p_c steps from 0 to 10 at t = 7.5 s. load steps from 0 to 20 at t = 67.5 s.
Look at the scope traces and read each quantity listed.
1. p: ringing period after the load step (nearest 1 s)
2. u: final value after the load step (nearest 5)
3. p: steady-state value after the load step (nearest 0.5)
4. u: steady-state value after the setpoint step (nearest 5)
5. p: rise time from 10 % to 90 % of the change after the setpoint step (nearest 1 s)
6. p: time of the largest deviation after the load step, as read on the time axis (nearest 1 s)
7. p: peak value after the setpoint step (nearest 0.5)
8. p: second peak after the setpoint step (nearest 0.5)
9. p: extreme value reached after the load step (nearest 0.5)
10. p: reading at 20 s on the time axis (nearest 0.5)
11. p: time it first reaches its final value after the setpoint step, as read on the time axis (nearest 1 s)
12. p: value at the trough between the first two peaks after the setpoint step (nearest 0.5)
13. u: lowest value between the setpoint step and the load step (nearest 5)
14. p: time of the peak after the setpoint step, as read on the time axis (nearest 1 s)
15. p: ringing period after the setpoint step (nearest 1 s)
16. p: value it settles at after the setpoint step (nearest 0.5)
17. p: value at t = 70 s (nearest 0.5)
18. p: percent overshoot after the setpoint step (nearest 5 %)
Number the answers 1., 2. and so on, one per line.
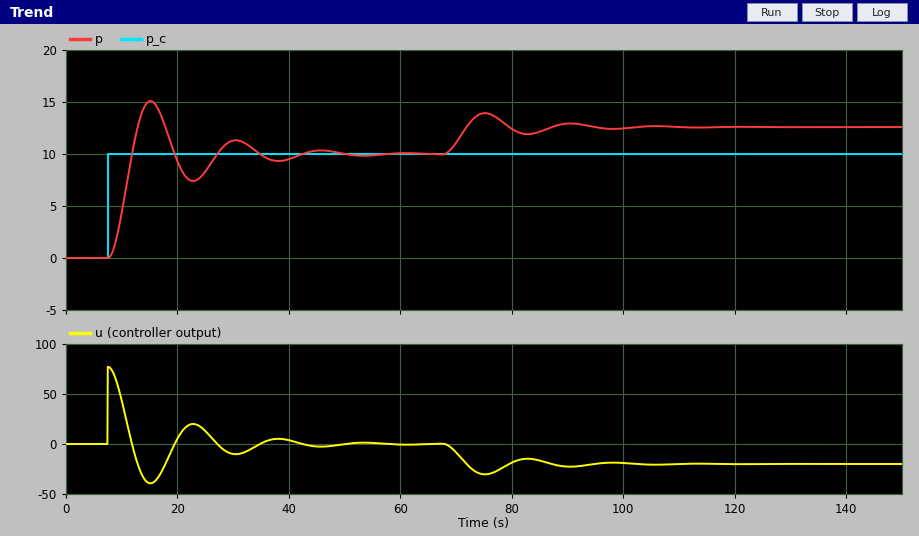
1. 15 s
2. -20
3. 12.5
4. 0
5. 3 s
6. 75 s
7. 15.0
8. 11.5
9. 14.0
10. 9.5
11. 12 s
12. 7.5
13. -40
14. 15 s
15. 15 s
16. 10.0
17. 11.0
18. 50 %
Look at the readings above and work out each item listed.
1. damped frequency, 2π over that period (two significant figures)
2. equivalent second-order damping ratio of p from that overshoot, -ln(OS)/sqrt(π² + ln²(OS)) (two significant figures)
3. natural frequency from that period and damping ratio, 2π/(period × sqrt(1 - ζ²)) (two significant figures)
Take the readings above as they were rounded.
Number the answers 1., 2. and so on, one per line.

1. 0.42 rad/s
2. 0.22
3. 0.43 rad/s
